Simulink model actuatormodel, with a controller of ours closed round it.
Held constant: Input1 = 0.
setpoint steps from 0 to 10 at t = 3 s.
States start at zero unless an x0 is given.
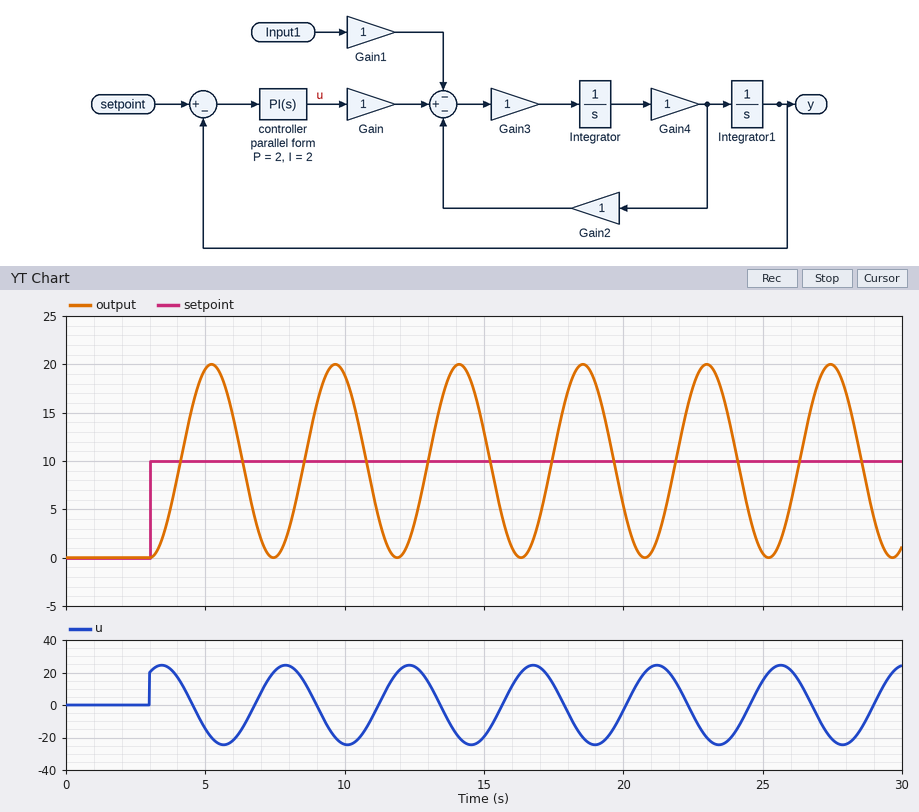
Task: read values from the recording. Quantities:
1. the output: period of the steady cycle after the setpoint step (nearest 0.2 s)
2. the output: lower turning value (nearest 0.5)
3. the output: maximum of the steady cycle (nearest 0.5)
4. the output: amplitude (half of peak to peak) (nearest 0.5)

4.4 s
0.0
20.0
10.0
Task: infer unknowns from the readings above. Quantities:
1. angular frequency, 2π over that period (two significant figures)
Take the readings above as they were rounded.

1.4 rad/s
